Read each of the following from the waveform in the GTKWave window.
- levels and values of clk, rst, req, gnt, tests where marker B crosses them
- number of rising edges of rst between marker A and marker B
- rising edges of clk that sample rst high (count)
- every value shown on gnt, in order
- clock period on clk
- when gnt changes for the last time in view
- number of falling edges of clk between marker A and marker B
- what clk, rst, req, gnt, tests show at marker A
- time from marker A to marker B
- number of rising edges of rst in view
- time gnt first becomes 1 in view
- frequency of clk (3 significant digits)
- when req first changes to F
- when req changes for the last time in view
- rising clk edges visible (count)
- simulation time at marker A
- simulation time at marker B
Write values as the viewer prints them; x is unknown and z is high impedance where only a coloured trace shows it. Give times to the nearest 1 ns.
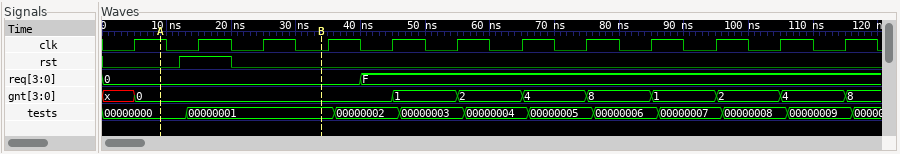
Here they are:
clk=0, rst=0, req=0, gnt=0, tests=00000001
1
1
x, 0, 1, 2, 4, 8, 1, 2, 4, 8
10 ns
115 ns
3
clk=1, rst=0, req=0, gnt=0, tests=00000000
25 ns
1
45 ns
100 MHz
40 ns
40 ns
12
9 ns
34 ns
